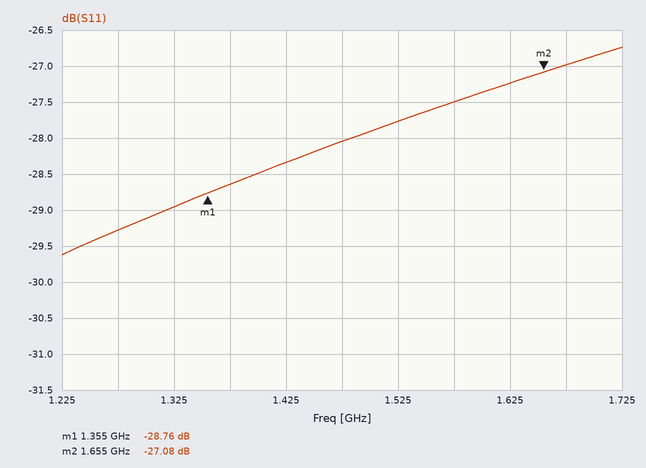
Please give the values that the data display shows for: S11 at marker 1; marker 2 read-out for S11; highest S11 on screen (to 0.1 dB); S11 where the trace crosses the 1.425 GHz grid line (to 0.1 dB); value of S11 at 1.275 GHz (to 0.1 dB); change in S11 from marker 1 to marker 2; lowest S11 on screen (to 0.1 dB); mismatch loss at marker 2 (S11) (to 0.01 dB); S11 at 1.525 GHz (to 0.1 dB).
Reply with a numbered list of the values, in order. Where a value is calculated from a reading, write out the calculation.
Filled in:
1. -28.76 dB
2. -27.08 dB
3. -26.7 dB
4. -28.3 dB
5. -29.3 dB
6. -27.08 − (-28.76) = 1.68 dB
7. -29.6 dB
8. −10 log10(1 − 10^(-27.08/10)) ≈ 0.01 dB
9. -27.8 dB
